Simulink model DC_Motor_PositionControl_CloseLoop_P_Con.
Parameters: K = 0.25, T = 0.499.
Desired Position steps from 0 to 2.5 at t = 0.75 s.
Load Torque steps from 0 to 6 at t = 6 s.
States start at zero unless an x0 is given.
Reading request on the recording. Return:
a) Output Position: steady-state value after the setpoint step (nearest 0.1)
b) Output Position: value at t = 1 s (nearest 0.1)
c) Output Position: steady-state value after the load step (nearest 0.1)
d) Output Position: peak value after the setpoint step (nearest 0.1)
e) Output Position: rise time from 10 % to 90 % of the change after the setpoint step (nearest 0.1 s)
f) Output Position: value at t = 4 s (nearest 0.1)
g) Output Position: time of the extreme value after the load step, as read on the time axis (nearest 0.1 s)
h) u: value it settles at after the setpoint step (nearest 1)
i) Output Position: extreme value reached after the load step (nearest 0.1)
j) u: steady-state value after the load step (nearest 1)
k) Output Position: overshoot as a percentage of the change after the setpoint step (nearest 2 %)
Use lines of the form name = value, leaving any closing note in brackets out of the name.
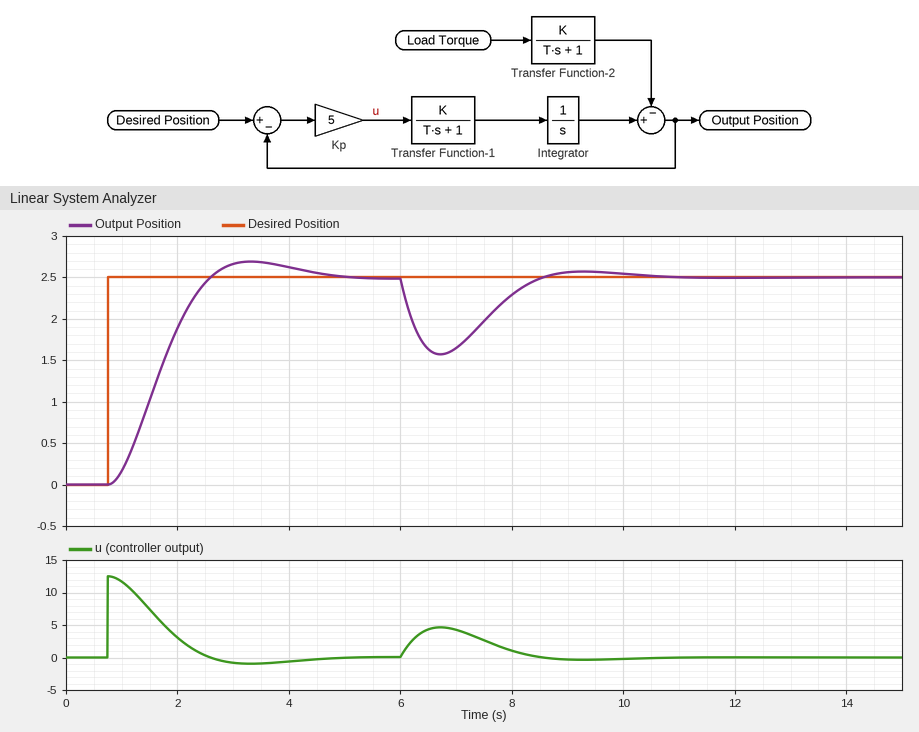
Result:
Output Position: steady-state value after the setpoint step = 2.5
Output Position: value at t = 1 s = 0.2
Output Position: steady-state value after the load step = 2.5
Output Position: peak value after the setpoint step = 2.7
Output Position: rise time from 10 % to 90 % of the change after the setpoint step = 1.2 s
Output Position: value at t = 4 s = 2.6
Output Position: time of the extreme value after the load step, as read on the time axis = 6.7 s
u: value it settles at after the setpoint step = 0
Output Position: extreme value reached after the load step = 1.6
u: steady-state value after the load step = 0
Output Position: overshoot as a percentage of the change after the setpoint step = 8 %
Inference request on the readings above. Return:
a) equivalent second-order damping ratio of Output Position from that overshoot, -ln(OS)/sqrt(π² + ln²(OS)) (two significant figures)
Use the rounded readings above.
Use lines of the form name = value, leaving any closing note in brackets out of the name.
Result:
equivalent second-order damping ratio of Output Position from that overshoot, -ln(OS)/sqrt(π² + ln²(OS)) = 0.63
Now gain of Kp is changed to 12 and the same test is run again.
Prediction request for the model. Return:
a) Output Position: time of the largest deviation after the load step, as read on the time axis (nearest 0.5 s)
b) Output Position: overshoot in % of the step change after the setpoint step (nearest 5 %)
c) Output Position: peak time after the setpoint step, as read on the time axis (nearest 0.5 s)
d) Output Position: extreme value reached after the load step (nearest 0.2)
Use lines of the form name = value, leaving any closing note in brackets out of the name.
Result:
Output Position: time of the largest deviation after the load step, as read on the time axis = 6.5 s
Output Position: overshoot in % of the step change after the setpoint step = 25 %
Output Position: peak time after the setpoint step, as read on the time axis = 2.0 s
Output Position: extreme value reached after the load step = 1.8
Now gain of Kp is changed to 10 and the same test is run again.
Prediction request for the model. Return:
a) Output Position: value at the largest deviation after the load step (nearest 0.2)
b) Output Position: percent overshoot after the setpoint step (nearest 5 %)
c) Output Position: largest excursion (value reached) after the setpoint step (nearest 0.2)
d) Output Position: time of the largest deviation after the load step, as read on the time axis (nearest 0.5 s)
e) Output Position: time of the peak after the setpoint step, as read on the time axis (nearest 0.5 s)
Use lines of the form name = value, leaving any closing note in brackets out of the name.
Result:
Output Position: value at the largest deviation after the load step = 1.8
Output Position: percent overshoot after the setpoint step = 20 %
Output Position: largest excursion (value reached) after the setpoint step = 3.0
Output Position: time of the largest deviation after the load step, as read on the time axis = 6.5 s
Output Position: time of the peak after the setpoint step, as read on the time axis = 2.5 s
